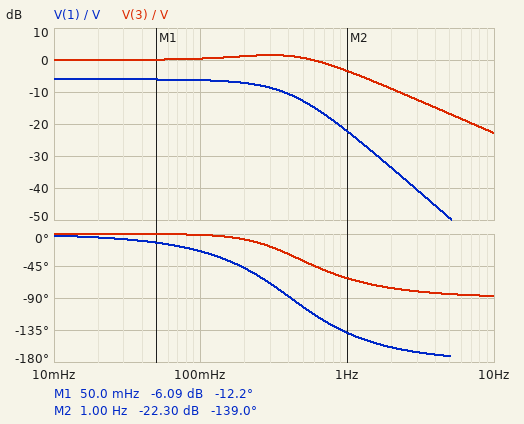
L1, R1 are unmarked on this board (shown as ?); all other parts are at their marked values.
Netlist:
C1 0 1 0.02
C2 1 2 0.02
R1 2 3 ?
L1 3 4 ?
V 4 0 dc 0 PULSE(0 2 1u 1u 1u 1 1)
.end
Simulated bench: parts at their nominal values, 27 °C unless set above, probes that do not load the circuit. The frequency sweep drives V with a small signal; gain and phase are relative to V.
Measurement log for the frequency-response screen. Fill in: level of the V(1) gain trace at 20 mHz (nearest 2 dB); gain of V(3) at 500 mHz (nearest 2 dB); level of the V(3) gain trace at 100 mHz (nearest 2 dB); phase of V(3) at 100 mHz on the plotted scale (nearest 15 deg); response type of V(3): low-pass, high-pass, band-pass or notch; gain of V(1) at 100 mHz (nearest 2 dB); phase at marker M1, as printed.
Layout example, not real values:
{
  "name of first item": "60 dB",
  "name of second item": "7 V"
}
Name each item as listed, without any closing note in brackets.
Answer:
{
  "level of the V(1) gain trace at 20 mHz": "-6 dB",
  "gain of V(3) at 500 mHz": "0 dB",
  "level of the V(3) gain trace at 100 mHz": "0 dB",
  "phase of V(3) at 100 mHz on the plotted scale": "0 deg",
  "response type of V(3): low-pass, high-pass, band-pass or notch": "low-pass",
  "gain of V(1) at 100 mHz": "-6 dB",
  "phase at marker M1, as printed": "-12.2 deg"
}
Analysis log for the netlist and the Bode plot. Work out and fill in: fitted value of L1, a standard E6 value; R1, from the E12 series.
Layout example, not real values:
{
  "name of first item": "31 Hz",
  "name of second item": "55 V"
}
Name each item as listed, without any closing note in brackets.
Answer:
{
  "fitted value of L1, a standard E6 value": "15 H",
  "R1, from the E12 series": "68 Ω"
}
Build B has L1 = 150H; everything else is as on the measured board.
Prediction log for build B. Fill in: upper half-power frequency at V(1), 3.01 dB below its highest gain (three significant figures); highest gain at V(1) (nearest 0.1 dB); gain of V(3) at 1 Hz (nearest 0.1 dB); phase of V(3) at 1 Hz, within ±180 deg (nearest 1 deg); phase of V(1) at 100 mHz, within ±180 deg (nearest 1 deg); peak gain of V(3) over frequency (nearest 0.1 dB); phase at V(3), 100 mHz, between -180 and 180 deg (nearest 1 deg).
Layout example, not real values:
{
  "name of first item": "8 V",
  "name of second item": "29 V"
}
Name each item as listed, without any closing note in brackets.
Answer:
{
  "upper half-power frequency at V(1), 3.01 dB below its highest gain": "153 mHz",
  "highest gain at V(1)": "-0.6 dB",
  "gain of V(3) at 1 Hz": "-22.5 dB",
  "phase of V(3) at 1 Hz, within ±180 deg": "-99 deg",
  "phase of V(1) at 100 mHz, within ±180 deg": "-46 deg",
  "peak gain of V(3) over frequency": "6.5 dB",
  "phase at V(3), 100 mHz, between -180 and 180 deg": "-23 deg"
}
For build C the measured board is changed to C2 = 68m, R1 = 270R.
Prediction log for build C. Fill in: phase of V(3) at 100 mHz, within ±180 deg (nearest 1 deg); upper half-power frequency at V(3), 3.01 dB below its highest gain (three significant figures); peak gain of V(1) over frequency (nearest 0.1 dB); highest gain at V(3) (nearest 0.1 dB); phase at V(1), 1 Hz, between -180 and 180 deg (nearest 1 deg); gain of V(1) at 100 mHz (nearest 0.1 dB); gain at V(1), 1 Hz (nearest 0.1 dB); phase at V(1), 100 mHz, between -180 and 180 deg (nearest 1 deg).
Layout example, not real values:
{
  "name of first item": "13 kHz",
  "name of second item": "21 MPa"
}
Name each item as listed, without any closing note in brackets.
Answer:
{
  "phase of V(3) at 100 mHz, within ±180 deg": "-2 deg",
  "upper half-power frequency at V(3), 3.01 dB below its highest gain": "2.84 Hz",
  "peak gain of V(1) over frequency": "-2.2 dB",
  "highest gain at V(3)": "0.1 dB",
  "phase at V(1), 1 Hz, between -180 and 180 deg": "-107 deg",
  "gain of V(1) at 100 mHz": "-11.1 dB",
  "gain at V(1), 1 Hz": "-31.0 dB",
  "phase at V(1), 100 mHz, between -180 and 180 deg": "-71 deg"
}
